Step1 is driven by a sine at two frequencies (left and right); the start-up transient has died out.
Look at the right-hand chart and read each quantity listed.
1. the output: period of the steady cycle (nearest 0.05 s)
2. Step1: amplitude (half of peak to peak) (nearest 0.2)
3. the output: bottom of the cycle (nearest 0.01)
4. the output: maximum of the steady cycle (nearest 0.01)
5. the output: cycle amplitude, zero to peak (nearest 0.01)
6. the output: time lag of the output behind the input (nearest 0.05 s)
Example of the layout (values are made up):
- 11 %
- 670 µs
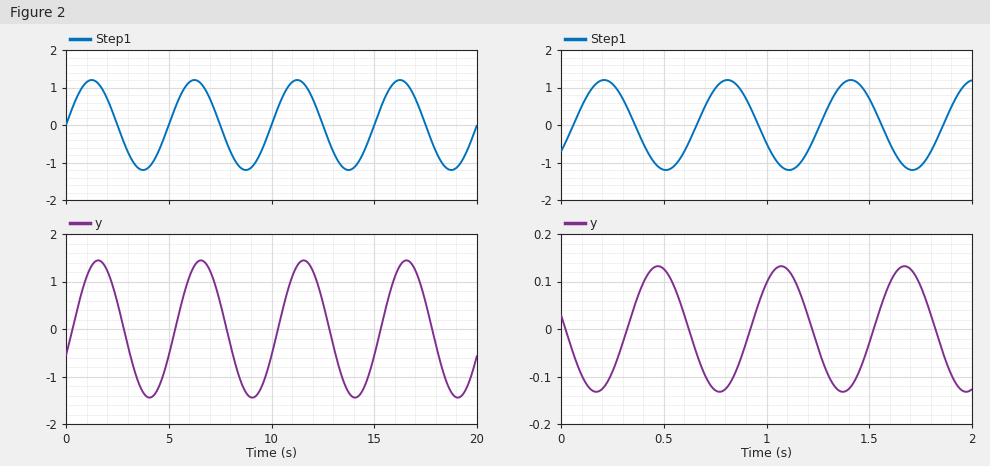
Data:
- 0.60 s
- 1.2
- -0.13
- 0.13
- 0.13
- 0.25 s
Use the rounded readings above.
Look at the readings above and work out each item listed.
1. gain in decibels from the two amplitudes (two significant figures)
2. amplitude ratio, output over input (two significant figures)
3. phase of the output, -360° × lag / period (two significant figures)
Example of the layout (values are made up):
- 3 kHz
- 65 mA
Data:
- -19 dB
- 0.11
- -150°
